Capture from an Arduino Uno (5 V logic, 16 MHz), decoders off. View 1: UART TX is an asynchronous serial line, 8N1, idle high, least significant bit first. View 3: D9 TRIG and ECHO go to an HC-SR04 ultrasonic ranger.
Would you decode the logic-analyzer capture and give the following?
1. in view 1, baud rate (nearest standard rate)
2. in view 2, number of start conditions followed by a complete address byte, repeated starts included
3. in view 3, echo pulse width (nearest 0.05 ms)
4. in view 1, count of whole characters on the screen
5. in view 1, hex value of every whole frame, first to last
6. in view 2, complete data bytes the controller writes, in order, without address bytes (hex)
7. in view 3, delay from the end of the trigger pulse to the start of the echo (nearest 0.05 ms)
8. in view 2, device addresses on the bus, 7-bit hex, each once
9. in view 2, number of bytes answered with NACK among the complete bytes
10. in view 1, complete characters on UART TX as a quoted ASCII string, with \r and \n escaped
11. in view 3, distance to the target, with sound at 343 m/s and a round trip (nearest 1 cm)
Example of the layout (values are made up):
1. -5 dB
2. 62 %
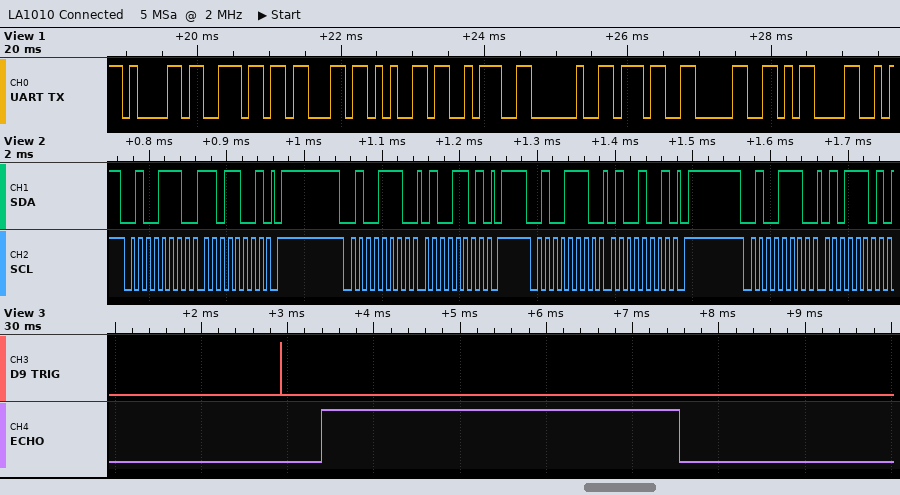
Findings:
1. 9600 baud
2. 4
3. 4.15 ms
4. 9
5. 61 6E 63 65 3A 20 37 30 0D
6. D9 4D 49 5D
7. 0.45 ms
8. 0x27
9. 0
10. "ance: 70\r"
11. 71 cm
